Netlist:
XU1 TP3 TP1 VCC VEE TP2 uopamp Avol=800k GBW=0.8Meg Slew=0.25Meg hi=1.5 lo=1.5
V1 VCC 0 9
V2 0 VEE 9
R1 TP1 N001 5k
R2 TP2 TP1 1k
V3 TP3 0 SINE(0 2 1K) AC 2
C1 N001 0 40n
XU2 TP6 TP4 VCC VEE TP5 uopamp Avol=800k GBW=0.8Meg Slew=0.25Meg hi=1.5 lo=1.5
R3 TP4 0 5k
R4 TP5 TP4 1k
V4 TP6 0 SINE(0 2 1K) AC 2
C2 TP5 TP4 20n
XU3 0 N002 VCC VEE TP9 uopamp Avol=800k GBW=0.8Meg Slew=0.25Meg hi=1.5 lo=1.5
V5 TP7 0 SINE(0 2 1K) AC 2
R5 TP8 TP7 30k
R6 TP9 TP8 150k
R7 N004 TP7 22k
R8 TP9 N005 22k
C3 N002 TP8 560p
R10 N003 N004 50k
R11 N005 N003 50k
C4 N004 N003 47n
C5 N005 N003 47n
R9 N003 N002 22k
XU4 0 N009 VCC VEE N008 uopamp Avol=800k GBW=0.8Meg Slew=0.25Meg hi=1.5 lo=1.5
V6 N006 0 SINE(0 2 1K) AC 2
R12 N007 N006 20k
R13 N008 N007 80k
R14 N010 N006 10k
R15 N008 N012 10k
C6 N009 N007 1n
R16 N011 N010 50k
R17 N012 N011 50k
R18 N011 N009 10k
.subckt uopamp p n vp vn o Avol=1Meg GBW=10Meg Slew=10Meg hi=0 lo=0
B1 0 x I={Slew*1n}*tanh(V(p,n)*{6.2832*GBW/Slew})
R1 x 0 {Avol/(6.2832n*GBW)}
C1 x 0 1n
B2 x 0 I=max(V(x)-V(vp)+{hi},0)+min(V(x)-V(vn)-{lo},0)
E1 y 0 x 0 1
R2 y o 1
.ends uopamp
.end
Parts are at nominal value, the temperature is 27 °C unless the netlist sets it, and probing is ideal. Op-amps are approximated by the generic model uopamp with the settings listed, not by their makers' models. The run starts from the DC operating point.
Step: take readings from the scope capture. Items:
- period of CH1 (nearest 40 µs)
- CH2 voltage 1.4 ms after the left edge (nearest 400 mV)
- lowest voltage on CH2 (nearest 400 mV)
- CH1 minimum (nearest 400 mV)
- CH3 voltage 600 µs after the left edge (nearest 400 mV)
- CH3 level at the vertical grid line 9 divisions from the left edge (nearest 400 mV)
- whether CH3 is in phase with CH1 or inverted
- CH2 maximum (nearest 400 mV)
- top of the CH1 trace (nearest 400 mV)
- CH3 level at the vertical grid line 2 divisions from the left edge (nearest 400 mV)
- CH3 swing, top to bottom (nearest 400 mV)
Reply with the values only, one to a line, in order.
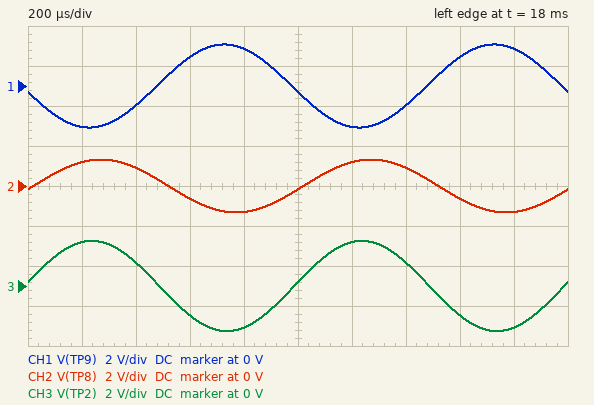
1.00 ms
800 mV
-1.2 V
-2.0 V
-1.6 V
-2.0 V
inverted
1.2 V
2.0 V
1.2 V
4.4 V
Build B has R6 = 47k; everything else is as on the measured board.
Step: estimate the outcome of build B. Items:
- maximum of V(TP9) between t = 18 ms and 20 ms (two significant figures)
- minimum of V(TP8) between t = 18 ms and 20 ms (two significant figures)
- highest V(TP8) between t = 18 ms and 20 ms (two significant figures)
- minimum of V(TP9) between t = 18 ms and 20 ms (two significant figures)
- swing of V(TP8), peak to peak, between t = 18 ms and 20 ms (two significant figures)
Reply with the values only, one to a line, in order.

2.0 V
-430 mV
430 mV
-2.0 V
870 mV
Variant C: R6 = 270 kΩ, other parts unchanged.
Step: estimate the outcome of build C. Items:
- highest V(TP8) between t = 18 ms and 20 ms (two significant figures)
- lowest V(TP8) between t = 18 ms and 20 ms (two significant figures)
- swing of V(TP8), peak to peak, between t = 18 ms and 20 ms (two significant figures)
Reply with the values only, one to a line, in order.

1.6 V
-1.6 V
3.2 V
